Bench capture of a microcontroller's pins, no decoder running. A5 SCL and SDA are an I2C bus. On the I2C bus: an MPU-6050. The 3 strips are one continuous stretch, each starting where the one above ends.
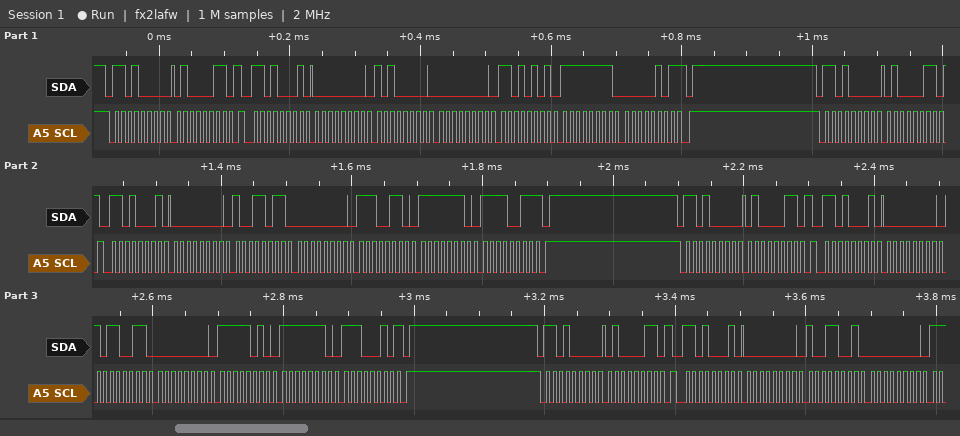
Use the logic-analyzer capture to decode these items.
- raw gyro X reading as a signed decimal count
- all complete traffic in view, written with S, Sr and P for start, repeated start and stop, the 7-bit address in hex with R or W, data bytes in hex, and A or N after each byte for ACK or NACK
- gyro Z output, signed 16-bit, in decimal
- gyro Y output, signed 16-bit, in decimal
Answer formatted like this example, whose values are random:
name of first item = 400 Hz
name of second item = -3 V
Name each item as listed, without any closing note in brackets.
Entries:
raw gyro X reading as a signed decimal count = 160
all complete traffic in view, written with S, Sr and P for start, repeated start and stop, the 7-bit address in hex with R or W, data bytes in hex, and A or N after each byte for ACK or NACK = S 68W A 43 A Sr 68R A 00 A A0 A 00 A D5 A FF A 05 N P S 68W A 43 A Sr 68R A 00 A 9B A 00 A E6 A FE A F3 N P S 68W A 43 A Sr 68R A 00 A B3 A 00 A FA A FE A E2 N P S 68W A 43 A Sr 68R A 00 A 99 A 00 A
gyro Z output, signed 16-bit, in decimal = -251
gyro Y output, signed 16-bit, in decimal = 213
